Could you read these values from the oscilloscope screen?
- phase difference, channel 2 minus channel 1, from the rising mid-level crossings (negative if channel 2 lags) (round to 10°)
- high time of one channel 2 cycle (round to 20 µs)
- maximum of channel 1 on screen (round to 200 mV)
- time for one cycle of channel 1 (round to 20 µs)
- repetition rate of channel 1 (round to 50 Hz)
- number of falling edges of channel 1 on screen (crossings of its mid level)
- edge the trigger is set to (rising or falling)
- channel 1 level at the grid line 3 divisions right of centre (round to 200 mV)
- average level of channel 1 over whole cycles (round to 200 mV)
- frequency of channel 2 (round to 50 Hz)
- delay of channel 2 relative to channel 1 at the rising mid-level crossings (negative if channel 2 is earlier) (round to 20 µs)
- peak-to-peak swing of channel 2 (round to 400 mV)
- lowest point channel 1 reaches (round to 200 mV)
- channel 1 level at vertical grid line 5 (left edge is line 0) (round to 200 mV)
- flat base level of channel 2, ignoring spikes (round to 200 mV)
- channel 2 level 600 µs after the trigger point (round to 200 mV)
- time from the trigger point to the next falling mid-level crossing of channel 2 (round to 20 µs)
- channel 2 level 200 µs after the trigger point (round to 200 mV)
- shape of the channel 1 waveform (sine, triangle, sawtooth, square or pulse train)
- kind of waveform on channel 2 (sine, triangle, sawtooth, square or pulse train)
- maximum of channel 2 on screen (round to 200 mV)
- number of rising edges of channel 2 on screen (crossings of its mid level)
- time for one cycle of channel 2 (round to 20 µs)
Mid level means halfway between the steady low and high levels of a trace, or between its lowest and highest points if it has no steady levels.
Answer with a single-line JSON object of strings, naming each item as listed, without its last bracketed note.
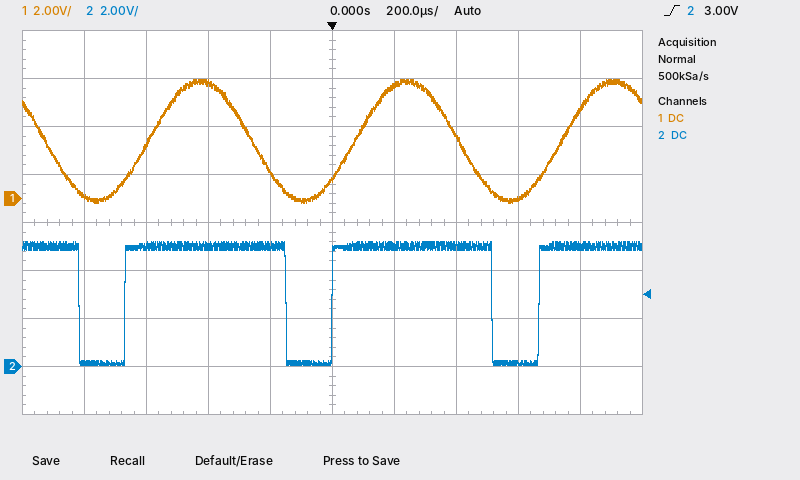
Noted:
{"phase difference, channel 2 minus channel 1, from the rising mid-level crossings (negative if channel 2 lags)": "+40°", "high time of one channel 2 cycle": "520 µs", "maximum of channel 1 on screen": "5.0 V", "time for one cycle of channel 1": "660 µs", "repetition rate of channel 1": "1.50 kHz", "number of falling edges of channel 1 on screen": "3", "edge the trigger is set to": "rising", "channel 1 level at the grid line 3 divisions right of centre": "0.0 V", "average level of channel 1 over whole cycles": "2.4 V", "frequency of channel 2": "1.50 kHz", "delay of channel 2 relative to channel 1 at the rising mid-level crossings (negative if channel 2 is earlier)": "-80 µs", "peak-to-peak swing of channel 2": "5.2 V", "lowest point channel 1 reaches": "-200 mV", "channel 1 level at vertical grid line 5 (left edge is line 0)": "800 mV", "flat base level of channel 2, ignoring spikes": "200 mV", "channel 2 level 600 µs after the trigger point": "200 mV", "time from the trigger point to the next falling mid-level crossing of channel 2": "520 µs", "channel 2 level 200 µs after the trigger point": "5.0 V", "shape of the channel 1 waveform": "sine", "kind of waveform on channel 2": "pulse train", "maximum of channel 2 on screen": "5.2 V", "number of rising edges of channel 2 on screen": "3", "time for one cycle of channel 2": "660 µs"}
